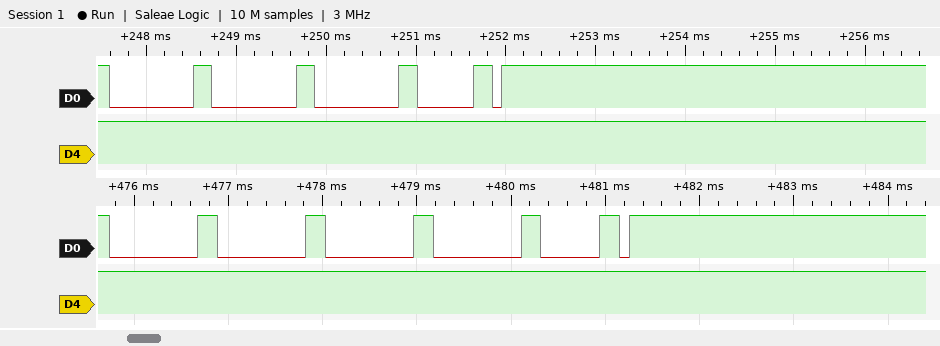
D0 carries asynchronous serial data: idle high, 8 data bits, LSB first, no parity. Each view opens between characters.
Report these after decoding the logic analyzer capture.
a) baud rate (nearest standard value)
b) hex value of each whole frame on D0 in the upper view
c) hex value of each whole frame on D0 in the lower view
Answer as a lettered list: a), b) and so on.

a) 9600 baud
b) 00, 00, 00, 60
c) 00, 00, 00, 00, 60
